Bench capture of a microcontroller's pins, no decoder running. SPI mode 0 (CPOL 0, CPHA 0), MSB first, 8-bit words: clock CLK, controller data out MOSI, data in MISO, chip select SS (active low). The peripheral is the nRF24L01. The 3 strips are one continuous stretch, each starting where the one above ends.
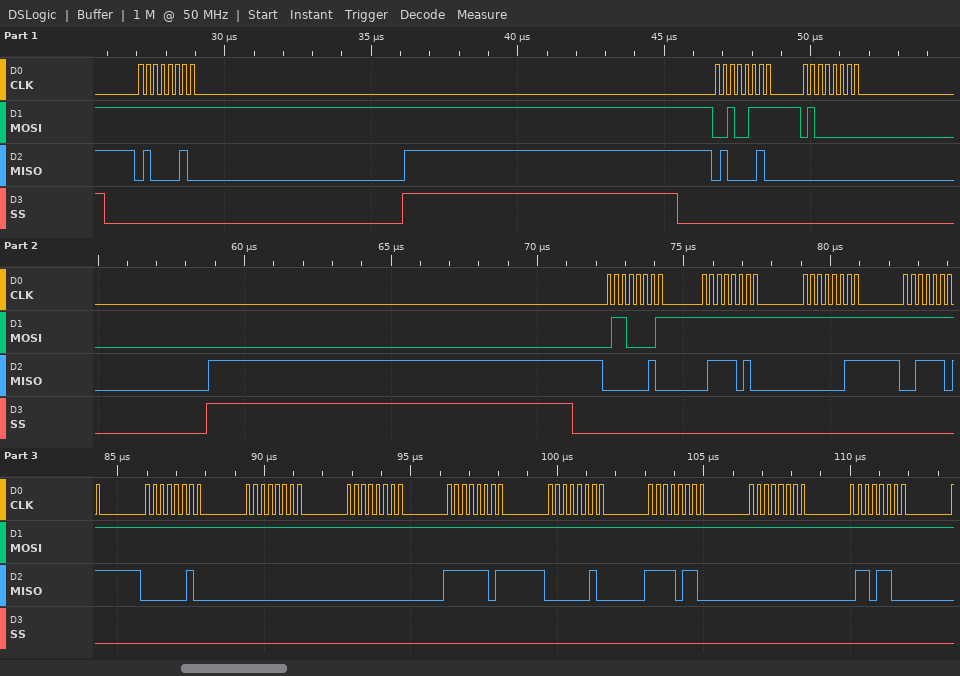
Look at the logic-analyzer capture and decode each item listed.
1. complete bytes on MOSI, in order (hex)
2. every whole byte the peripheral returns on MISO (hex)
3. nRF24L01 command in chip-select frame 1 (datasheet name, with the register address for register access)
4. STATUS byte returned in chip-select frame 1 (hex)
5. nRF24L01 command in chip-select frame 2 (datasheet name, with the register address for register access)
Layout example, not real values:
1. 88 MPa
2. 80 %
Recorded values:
1. FF 27 40 61 FF FF FF FF FF FF FF FF FF FF FF
2. 42 42 00 02 7A 03 3D 02 00 00 FD 02 F6 00 6C
3. NOP
4. 0x42
5. W_REGISTER 0x07
